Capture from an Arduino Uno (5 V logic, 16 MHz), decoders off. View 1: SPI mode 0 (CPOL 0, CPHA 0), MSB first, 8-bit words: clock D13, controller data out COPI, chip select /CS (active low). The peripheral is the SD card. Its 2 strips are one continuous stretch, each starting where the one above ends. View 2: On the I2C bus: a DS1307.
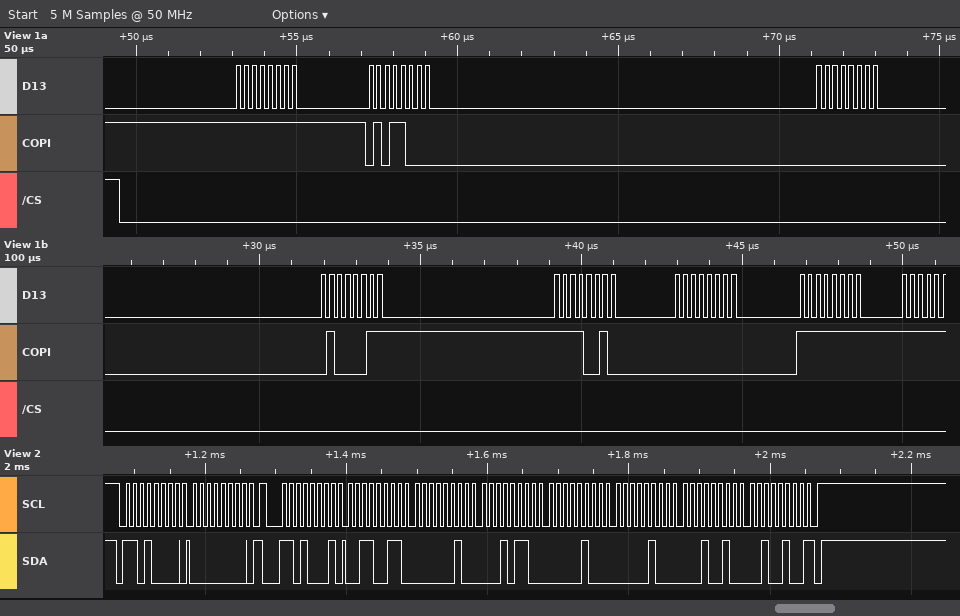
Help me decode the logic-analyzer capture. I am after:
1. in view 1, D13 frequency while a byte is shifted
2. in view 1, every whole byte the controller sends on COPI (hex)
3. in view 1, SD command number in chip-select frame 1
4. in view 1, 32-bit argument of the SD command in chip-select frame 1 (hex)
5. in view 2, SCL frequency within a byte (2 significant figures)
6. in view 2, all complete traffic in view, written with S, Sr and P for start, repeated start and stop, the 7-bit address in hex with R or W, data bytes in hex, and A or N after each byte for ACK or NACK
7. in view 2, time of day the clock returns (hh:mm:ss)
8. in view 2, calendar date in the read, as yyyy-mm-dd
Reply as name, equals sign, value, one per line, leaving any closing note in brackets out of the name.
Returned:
in view 1, D13 frequency while a byte is shifted = 4 MHz
in view 1, every whole byte the controller sends on COPI = FF 58 00 43 F2 00 FF
in view 1, SD command number in chip-select frame 1 = CMD24
in view 1, 32-bit argument of the SD command in chip-select frame 1 = 0x0043F200
in view 2, SCL frequency within a byte = 100 kHz
in view 2, all complete traffic in view, written with S, Sr and P for start, repeated start and stop, the 7-bit address in hex with R or W, data bytes in hex, and A or N after each byte for ACK or NACK = S 68W A 00 A Sr 68R A 33 A 02 A 16 A 04 A 04 A 12 A 24 N P
in view 2, time of day the clock returns = 16:02:33
in view 2, calendar date in the read, as yyyy-mm-dd = 2024-12-04
